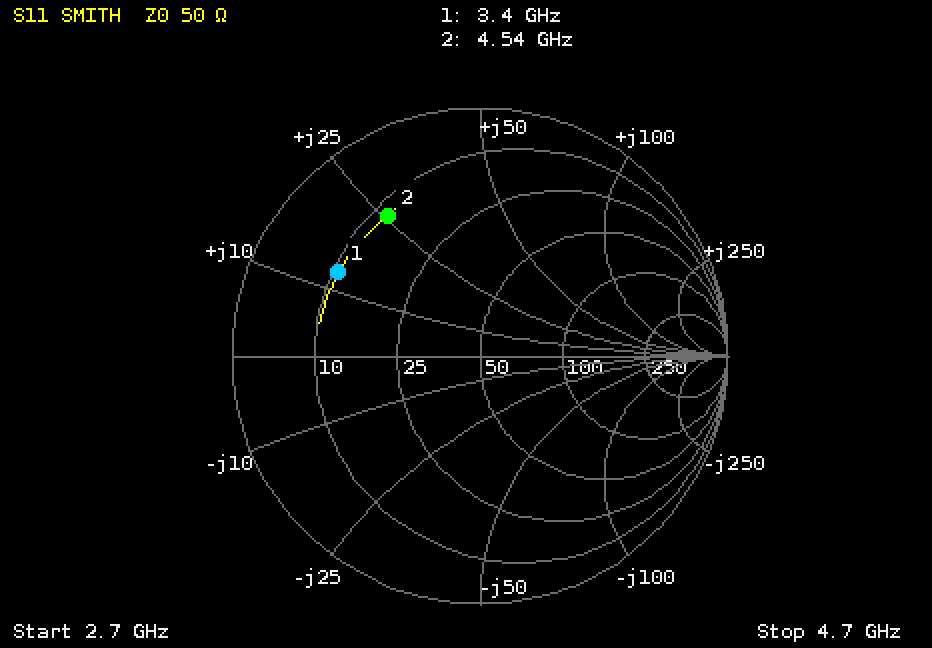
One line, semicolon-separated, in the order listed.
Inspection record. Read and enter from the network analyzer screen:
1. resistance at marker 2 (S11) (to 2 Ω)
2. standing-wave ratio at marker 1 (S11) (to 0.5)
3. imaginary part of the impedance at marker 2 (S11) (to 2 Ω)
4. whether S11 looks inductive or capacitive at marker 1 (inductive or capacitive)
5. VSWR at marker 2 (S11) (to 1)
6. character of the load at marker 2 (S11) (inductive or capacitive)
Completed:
12 Ω; 5.0; +26 Ω; inductive; 5; inductive
